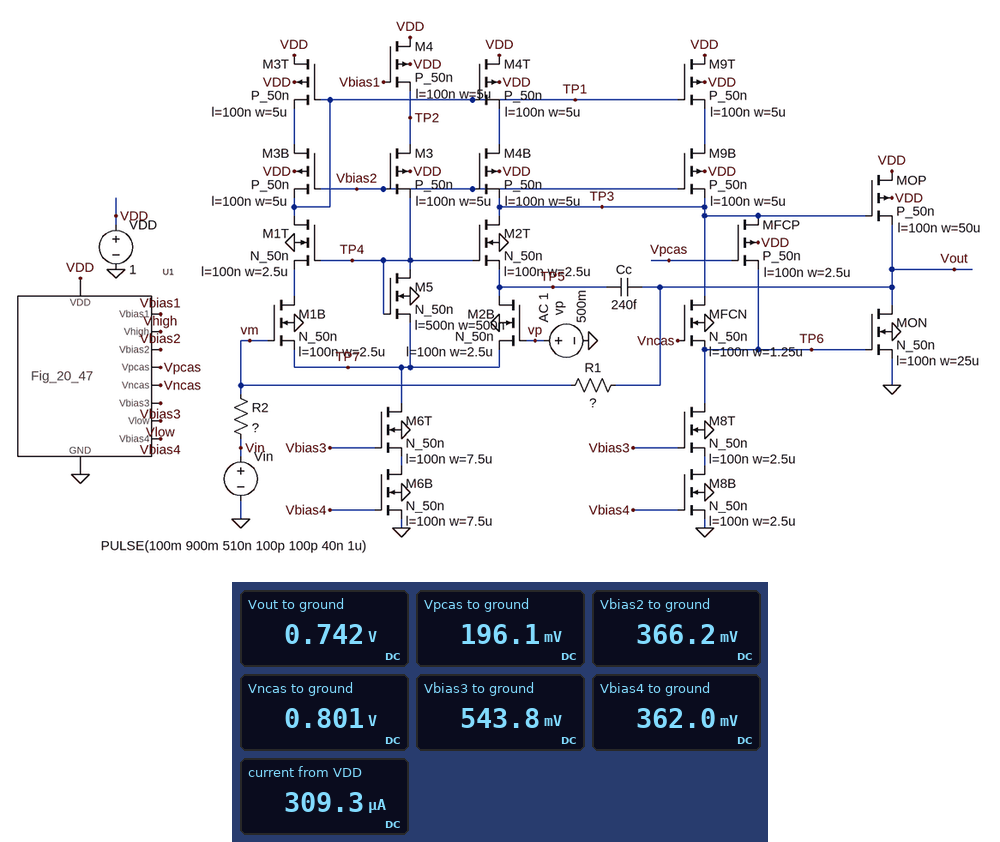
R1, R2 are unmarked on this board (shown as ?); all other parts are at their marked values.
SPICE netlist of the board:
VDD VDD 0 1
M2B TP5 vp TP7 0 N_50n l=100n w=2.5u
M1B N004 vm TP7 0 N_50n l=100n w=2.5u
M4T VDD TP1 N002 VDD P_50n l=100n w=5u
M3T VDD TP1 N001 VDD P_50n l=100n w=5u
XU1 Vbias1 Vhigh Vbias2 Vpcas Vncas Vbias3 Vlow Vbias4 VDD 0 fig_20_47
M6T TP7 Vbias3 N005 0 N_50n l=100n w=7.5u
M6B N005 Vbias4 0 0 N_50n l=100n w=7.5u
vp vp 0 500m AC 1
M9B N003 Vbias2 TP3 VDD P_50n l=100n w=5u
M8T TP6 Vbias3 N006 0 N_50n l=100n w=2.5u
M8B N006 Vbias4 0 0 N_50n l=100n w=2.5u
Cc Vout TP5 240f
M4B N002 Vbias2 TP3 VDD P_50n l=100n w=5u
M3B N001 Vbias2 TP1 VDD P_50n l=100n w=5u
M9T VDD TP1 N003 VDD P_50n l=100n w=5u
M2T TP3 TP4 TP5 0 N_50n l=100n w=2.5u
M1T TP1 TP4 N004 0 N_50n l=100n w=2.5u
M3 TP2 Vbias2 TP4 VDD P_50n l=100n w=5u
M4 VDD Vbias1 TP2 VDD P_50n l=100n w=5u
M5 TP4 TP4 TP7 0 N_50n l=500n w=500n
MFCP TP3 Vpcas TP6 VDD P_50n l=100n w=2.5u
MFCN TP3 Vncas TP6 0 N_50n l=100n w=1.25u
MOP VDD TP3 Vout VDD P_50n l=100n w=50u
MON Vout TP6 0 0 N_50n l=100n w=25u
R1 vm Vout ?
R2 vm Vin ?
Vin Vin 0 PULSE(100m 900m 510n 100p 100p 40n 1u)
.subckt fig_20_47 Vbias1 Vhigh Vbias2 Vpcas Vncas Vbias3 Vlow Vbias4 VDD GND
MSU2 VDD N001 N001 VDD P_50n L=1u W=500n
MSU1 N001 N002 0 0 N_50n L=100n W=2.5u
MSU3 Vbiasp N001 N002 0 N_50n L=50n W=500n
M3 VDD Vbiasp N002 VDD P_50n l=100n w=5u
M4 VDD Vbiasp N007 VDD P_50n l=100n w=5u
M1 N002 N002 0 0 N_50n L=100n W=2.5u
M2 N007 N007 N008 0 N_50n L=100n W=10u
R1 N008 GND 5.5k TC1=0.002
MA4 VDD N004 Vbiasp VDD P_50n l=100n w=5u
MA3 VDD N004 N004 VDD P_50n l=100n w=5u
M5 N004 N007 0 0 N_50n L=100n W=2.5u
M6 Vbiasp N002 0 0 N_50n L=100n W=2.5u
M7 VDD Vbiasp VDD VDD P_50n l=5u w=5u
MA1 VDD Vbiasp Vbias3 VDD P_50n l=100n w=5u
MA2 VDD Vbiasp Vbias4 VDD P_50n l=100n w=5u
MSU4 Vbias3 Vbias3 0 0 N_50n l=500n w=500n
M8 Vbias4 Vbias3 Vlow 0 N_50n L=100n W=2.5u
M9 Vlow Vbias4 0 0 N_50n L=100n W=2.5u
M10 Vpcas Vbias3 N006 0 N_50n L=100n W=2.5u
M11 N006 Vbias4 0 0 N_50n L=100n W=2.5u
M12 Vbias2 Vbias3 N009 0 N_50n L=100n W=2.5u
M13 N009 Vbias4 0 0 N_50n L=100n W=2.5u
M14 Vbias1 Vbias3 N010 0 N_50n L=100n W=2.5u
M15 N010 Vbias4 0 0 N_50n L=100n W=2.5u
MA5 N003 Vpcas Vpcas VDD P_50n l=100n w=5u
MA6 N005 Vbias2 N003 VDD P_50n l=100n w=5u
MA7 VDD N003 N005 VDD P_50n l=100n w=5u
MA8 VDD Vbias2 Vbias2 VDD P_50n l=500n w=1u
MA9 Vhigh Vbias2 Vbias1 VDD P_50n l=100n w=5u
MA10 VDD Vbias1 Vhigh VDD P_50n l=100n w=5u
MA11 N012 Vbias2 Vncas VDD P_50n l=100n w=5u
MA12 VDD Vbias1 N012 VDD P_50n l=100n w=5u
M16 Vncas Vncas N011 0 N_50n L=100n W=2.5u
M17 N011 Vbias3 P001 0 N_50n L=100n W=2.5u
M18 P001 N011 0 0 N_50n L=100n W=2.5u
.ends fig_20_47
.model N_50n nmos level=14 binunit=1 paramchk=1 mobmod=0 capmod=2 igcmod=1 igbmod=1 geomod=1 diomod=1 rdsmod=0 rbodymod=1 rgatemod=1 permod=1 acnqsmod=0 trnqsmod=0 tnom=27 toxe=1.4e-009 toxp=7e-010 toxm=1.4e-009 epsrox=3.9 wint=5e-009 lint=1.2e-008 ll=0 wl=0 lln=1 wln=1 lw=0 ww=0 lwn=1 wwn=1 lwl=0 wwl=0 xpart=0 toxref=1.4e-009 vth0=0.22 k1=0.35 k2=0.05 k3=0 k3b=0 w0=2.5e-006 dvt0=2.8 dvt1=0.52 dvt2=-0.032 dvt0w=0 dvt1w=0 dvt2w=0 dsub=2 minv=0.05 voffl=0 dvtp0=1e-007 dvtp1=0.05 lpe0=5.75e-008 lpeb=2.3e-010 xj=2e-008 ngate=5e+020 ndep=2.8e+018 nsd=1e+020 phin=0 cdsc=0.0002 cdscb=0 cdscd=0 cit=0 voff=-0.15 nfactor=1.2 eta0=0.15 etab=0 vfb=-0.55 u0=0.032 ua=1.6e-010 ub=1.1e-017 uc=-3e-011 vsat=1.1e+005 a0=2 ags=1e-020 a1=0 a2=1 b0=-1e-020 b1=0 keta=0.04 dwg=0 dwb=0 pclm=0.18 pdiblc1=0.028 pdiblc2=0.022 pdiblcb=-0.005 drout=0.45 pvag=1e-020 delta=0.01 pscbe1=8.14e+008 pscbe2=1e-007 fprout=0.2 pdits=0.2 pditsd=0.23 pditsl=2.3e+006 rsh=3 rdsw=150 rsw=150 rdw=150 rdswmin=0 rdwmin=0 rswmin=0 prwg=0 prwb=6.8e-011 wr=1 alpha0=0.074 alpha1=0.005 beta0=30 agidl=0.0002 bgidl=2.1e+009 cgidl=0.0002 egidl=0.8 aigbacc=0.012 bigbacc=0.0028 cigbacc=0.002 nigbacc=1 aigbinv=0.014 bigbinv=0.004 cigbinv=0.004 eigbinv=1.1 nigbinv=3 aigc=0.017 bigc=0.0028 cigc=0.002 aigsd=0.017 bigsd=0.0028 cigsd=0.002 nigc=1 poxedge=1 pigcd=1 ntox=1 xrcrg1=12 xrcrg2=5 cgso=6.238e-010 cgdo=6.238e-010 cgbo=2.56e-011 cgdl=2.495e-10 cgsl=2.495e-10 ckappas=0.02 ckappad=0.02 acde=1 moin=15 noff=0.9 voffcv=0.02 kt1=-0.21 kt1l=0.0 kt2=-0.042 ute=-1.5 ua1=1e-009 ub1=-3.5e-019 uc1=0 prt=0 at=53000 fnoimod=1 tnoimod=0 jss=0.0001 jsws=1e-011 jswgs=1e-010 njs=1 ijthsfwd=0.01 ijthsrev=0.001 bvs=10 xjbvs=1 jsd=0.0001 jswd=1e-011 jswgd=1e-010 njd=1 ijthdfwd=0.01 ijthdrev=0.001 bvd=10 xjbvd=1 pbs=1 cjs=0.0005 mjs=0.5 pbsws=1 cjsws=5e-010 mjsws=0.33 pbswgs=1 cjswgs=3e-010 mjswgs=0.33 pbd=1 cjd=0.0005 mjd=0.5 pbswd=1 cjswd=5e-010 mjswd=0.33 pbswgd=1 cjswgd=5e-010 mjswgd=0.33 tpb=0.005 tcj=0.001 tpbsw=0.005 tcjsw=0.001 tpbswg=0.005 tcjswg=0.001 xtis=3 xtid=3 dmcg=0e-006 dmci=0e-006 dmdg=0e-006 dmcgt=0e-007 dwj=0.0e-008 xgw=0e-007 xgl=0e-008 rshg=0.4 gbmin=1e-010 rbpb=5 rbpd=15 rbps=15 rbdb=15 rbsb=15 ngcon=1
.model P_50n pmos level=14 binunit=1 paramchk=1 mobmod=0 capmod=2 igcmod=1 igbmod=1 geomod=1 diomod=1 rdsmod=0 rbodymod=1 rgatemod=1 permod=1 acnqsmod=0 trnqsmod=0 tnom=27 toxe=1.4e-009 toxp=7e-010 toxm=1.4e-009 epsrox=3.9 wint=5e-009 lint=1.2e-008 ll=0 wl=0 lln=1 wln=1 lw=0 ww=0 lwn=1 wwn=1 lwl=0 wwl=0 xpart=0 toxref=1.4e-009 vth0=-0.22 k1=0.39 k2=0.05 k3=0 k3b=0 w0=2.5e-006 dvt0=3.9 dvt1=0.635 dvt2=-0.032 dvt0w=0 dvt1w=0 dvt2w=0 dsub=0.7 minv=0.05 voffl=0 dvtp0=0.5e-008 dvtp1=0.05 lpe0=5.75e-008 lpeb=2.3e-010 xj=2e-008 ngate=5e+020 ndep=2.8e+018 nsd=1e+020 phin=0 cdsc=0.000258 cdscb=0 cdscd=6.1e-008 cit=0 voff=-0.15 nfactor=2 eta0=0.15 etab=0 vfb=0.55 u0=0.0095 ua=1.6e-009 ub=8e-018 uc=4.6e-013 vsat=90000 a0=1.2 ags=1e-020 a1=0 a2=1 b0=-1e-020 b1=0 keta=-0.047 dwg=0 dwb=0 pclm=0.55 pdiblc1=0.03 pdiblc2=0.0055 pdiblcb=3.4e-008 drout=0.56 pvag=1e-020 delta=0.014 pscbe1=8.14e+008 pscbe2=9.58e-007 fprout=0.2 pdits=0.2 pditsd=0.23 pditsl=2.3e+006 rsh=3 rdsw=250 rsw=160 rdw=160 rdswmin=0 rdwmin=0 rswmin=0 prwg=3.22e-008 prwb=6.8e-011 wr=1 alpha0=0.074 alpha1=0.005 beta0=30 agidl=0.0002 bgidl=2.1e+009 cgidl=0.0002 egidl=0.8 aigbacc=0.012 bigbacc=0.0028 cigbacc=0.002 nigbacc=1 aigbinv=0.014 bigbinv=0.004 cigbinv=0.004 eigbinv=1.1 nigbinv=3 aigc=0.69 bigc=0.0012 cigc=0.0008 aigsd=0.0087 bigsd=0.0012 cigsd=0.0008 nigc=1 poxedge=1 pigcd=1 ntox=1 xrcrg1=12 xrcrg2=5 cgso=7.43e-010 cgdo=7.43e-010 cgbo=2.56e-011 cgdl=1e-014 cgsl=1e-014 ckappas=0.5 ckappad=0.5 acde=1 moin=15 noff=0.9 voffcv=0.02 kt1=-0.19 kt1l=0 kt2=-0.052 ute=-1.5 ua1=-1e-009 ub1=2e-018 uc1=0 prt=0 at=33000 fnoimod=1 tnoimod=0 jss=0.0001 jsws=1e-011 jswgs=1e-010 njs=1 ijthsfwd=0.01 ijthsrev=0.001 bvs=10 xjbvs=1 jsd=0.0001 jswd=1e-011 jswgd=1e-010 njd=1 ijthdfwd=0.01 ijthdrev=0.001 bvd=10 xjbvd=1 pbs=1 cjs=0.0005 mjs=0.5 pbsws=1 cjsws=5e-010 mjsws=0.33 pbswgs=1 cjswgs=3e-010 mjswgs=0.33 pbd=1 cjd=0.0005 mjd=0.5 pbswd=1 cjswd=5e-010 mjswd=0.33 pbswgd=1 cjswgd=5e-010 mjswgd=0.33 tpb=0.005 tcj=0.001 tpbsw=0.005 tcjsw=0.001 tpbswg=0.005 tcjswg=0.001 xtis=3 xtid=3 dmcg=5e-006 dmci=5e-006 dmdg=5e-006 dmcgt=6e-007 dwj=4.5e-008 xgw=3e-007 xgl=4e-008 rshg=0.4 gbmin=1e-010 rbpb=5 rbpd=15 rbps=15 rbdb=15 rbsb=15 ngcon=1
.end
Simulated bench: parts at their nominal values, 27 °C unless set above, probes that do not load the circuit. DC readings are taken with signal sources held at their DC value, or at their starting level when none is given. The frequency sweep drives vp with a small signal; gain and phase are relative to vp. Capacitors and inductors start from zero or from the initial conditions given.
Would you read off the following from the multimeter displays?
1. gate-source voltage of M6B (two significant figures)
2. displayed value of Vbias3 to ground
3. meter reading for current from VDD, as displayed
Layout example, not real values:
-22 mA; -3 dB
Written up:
360 mV; 543.8 mV; 309.3 µA
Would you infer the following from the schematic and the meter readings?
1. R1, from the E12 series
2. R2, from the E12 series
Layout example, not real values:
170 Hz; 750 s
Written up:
3.3 kΩ; 5.6 kΩ
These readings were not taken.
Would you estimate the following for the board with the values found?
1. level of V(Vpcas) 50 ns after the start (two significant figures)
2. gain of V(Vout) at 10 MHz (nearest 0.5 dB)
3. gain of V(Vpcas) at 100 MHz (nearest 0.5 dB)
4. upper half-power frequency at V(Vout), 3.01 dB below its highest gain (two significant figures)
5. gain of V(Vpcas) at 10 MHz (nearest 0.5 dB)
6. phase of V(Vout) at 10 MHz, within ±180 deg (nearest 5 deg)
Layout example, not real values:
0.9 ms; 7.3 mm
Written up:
250 mV; 3.5 dB; -31.5 dB; 330 MHz; -50.0 dB; -5 deg
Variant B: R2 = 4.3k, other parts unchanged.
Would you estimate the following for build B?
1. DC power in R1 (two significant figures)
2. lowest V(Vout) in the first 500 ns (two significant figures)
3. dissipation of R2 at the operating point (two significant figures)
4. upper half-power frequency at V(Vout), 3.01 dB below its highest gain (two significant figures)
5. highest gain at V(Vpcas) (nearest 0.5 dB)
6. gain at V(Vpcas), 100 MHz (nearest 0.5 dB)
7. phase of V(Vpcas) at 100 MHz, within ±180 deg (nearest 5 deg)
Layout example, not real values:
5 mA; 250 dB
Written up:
29 µW; 210 mV; 38 µW; 140 MHz; -30.0 dB; -32.0 dB; -170 deg
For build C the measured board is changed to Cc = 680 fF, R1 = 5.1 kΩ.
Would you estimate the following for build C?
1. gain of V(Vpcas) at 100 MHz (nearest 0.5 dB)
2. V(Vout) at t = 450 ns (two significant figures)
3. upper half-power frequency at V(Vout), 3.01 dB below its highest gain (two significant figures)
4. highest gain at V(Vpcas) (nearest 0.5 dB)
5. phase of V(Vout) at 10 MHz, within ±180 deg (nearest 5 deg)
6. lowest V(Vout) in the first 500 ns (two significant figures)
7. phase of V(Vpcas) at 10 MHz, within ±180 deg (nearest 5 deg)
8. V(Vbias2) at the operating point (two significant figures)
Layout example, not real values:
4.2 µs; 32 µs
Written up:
-34.0 dB; 870 mV; 40 MHz; -30.0 dB; -15 deg; 200 mV; -100 deg; 370 mV
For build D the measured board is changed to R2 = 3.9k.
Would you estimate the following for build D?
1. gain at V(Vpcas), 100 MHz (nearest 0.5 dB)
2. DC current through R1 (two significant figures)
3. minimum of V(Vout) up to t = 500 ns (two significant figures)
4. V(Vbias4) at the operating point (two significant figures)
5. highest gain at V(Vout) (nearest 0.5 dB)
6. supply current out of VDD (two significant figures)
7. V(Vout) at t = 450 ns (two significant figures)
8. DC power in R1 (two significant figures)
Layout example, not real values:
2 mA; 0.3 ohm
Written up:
-32.0 dB; 100 µA; 210 mV; 360 mV; 4.5 dB; 340 µA; 850 mV; 35 µW
